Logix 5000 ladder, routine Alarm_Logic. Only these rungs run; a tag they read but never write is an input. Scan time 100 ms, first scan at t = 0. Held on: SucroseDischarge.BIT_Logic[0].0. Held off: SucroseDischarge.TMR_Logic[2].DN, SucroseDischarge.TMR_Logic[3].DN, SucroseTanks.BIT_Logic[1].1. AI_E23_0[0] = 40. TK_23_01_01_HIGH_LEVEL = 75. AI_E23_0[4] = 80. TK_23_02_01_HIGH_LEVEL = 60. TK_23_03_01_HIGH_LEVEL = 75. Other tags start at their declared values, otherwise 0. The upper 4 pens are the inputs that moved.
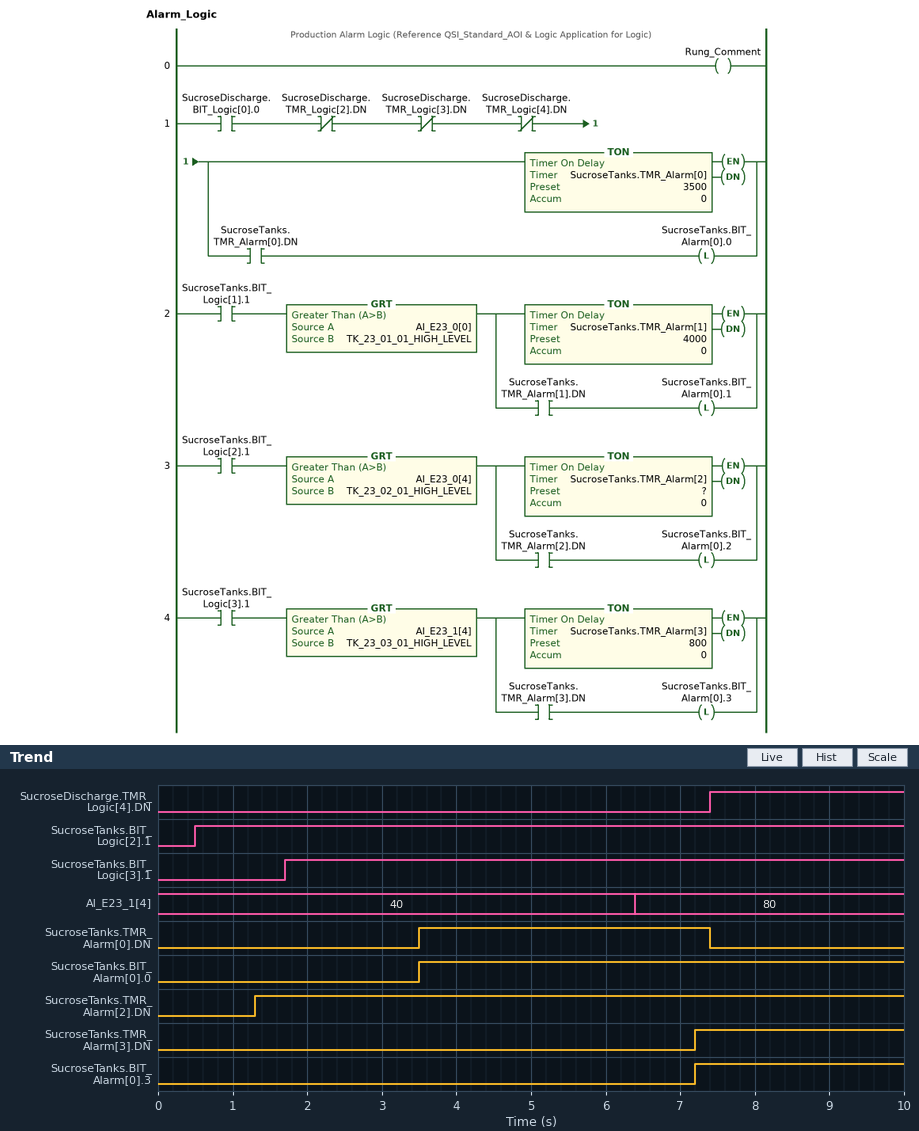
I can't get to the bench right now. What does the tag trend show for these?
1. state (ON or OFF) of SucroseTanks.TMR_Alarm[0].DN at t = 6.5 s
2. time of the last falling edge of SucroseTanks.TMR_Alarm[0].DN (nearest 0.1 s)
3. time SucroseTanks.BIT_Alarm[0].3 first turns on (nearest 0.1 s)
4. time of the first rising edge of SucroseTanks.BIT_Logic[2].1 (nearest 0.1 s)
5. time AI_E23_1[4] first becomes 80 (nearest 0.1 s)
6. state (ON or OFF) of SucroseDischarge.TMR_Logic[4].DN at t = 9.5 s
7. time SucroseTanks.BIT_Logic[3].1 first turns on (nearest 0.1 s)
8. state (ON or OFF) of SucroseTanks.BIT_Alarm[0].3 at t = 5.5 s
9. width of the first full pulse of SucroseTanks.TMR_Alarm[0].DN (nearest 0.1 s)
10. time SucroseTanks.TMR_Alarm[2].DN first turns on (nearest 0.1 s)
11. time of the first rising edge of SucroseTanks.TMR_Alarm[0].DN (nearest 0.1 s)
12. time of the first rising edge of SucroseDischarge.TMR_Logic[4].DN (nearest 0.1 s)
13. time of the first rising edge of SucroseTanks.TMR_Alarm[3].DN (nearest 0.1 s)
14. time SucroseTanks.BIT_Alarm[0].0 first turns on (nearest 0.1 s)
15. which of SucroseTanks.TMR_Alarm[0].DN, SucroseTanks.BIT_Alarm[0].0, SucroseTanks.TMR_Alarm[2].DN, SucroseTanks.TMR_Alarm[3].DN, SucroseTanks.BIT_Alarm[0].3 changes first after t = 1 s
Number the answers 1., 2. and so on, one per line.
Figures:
1. ON
2. 7.4 s
3. 7.2 s
4. 0.5 s
5. 6.4 s
6. ON
7. 1.7 s
8. OFF
9. 3.9 s
10. 1.3 s
11. 3.5 s
12. 7.4 s
13. 7.2 s
14. 3.5 s
15. SucroseTanks.TMR_Alarm[2].DN
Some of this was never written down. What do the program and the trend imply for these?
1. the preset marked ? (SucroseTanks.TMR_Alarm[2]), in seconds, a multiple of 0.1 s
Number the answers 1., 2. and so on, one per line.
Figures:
1. 0.8 s
